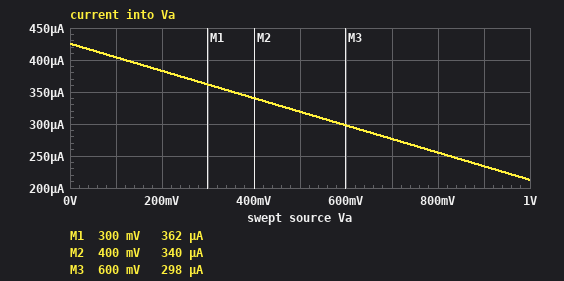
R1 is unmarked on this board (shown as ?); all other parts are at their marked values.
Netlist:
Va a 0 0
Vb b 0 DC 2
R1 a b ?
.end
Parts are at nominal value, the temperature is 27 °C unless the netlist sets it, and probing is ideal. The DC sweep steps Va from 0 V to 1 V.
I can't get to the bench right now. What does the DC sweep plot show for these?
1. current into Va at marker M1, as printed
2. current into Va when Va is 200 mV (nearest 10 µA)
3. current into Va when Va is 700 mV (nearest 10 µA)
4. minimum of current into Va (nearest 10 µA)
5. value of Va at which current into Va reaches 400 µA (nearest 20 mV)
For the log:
362 µA
380 µA
280 µA
210 µA
120 mV
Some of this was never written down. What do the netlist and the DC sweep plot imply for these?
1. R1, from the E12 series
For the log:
4.7 kΩ
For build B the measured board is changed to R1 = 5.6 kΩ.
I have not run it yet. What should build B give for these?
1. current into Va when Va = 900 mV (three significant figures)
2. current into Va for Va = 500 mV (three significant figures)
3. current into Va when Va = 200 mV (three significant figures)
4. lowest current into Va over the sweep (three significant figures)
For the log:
196 µA
268 µA
321 µA
179 µA
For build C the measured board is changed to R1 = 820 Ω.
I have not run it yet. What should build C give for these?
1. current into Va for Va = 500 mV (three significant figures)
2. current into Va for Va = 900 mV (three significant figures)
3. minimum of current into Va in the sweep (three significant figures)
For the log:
1.83 mA
1.34 mA
1.22 mA
